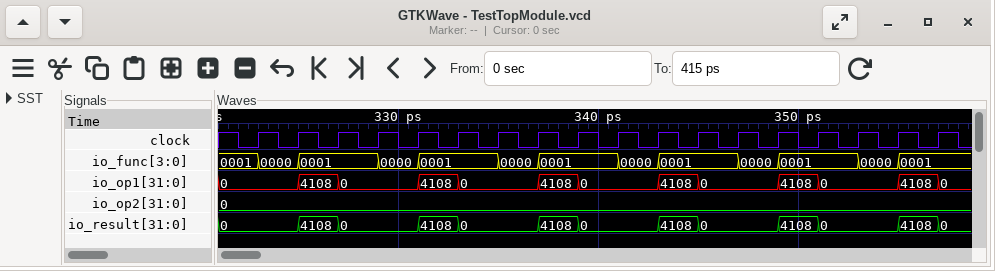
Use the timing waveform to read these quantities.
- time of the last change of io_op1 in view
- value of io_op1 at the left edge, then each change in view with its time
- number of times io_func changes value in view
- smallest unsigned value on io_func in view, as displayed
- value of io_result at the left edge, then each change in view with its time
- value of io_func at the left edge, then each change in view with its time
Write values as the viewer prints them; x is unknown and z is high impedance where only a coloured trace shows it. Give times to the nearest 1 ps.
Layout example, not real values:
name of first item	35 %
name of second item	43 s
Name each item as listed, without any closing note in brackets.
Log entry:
time of the last change of io_op1 in view	357 ps
value of io_op1 at the left edge, then each change in view with its time	0, 4108 at 325 ps, 0 at 327 ps, 4108 at 331 ps, 0 at 333 ps, 4108 at 337 ps, 0 at 339 ps, 4108 at 343 ps, 0 at 345 ps, 4108 at 349 ps, 0 at 351 ps, 4108 at 355 ps, 0 at 357 ps
number of times io_func changes value in view	12
smallest unsigned value on io_func in view, as displayed	0000
value of io_result at the left edge, then each change in view with its time	0, 4108 at 325 ps, 0 at 327 ps, 4108 at 331 ps, 0 at 333 ps, 4108 at 337 ps, 0 at 339 ps, 4108 at 343 ps, 0 at 345 ps, 4108 at 349 ps, 0 at 351 ps, 4108 at 355 ps, 0 at 357 ps
value of io_func at the left edge, then each change in view with its time	0001, 0000 at 323 ps, 0001 at 325 ps, 0000 at 329 ps, 0001 at 331 ps, 0000 at 335 ps, 0001 at 337 ps, 0000 at 341 ps, 0001 at 343 ps, 0000 at 347 ps, 0001 at 349 ps, 0000 at 353 ps, 0001 at 355 ps
